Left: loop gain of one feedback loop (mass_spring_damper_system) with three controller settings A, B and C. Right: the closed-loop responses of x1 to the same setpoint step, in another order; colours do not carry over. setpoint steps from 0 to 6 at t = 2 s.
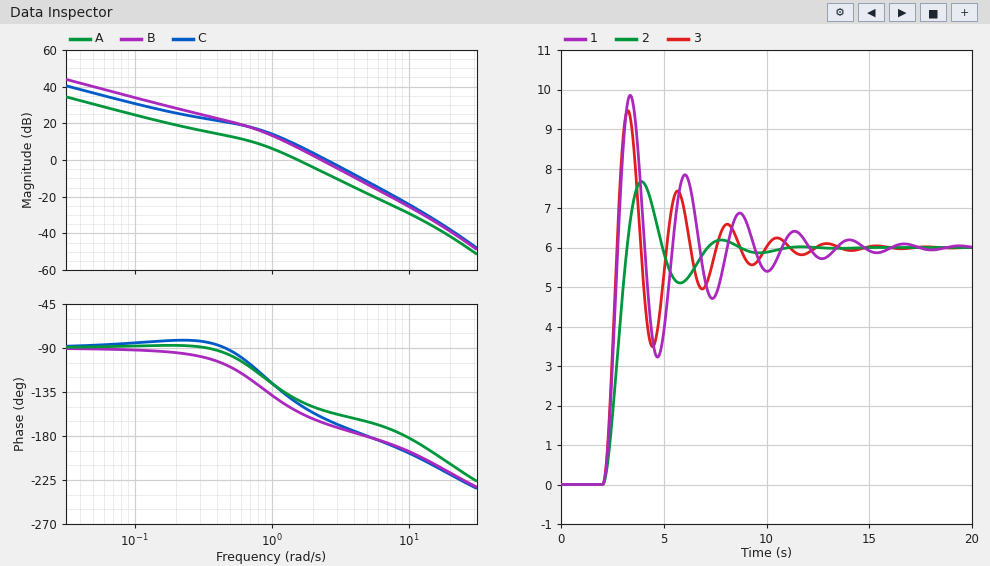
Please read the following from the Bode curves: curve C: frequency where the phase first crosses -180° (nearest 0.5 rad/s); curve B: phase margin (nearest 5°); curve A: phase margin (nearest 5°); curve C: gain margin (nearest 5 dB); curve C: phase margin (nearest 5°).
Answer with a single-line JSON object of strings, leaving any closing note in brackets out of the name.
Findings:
{"curve C: frequency where the phase first crosses -180°": "5.0 rad/s", "curve B: phase margin": "15°", "curve A: phase margin": "35°", "curve C: gain margin": "10 dB", "curve C: phase margin": "15°"}
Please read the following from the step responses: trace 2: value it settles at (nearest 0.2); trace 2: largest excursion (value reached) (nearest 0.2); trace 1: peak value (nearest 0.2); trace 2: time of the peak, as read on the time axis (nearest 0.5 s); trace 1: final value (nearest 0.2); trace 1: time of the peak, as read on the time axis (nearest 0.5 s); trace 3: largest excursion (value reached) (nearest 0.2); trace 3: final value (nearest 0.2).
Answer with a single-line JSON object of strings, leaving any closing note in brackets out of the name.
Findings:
{"trace 2: value it settles at": "6.0", "trace 2: largest excursion (value reached)": "7.6", "trace 1: peak value": "9.8", "trace 2: time of the peak, as read on the time axis": "4.0 s", "trace 1: final value": "6.0", "trace 1: time of the peak, as read on the time axis": "3.5 s", "trace 3: largest excursion (value reached)": "9.4", "trace 3: final value": "6.0"}
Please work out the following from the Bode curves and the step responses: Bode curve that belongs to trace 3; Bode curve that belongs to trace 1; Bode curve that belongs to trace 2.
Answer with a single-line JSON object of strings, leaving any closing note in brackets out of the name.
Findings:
{"Bode curve that belongs to trace 3": "C", "Bode curve that belongs to trace 1": "B", "Bode curve that belongs to trace 2": "A"}
